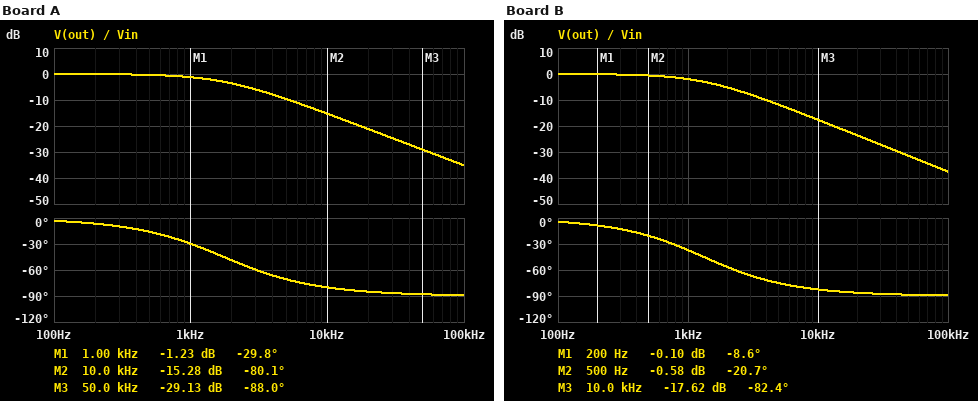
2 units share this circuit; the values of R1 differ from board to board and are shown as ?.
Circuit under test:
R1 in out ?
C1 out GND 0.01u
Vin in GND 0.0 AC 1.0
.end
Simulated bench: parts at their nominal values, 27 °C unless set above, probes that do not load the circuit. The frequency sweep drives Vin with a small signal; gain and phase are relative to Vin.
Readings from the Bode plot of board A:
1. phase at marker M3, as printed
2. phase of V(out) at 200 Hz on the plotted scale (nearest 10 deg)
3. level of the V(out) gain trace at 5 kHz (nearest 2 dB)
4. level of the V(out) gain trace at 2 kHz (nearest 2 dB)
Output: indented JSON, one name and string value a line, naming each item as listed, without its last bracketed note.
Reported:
{
  "phase at marker M3, as printed": "-88.0 deg",
  "phase of V(out) at 200 Hz on the plotted scale": "-10 deg",
  "level of the V(out) gain trace at 5 kHz": "-10 dB",
  "level of the V(out) gain trace at 2 kHz": "-4 dB"
}
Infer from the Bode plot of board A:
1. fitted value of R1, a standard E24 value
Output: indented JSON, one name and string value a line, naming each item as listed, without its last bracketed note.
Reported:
{
  "fitted value of R1, a standard E24 value": "9.1 kΩ"
}
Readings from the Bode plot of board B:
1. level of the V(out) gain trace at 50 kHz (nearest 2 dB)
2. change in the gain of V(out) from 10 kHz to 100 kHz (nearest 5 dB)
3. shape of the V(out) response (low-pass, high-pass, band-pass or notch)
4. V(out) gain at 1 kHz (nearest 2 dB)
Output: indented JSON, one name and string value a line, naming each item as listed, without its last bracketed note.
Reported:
{
  "level of the V(out) gain trace at 50 kHz": "-32 dB",
  "change in the gain of V(out) from 10 kHz to 100 kHz": "-20 dB",
  "shape of the V(out) response": "low-pass",
  "V(out) gain at 1 kHz": "-2 dB"
}
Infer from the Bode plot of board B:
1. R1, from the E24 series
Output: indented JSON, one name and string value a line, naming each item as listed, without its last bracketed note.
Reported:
{
  "R1, from the E24 series": "12 kΩ"
}
